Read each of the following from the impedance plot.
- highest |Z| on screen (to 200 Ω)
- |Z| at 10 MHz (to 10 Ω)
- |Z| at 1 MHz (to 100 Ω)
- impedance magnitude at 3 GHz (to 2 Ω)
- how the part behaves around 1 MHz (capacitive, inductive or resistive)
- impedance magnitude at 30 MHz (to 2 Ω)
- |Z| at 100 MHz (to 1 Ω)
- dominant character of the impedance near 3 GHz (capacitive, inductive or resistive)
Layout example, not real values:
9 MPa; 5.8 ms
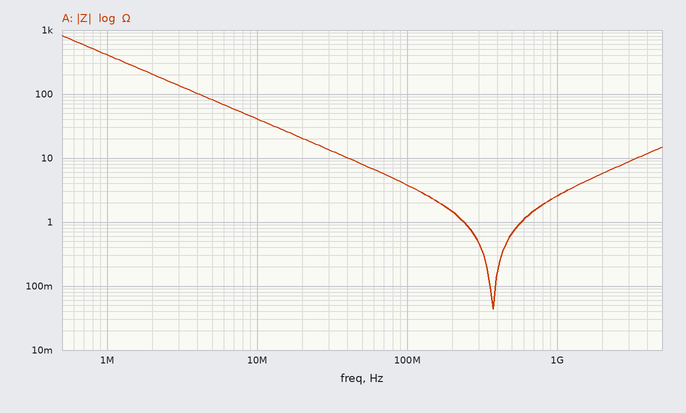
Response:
800 Ω; 40 Ω; 400 Ω; 8 Ω; capacitive; 14 Ω; 4 Ω; inductive
